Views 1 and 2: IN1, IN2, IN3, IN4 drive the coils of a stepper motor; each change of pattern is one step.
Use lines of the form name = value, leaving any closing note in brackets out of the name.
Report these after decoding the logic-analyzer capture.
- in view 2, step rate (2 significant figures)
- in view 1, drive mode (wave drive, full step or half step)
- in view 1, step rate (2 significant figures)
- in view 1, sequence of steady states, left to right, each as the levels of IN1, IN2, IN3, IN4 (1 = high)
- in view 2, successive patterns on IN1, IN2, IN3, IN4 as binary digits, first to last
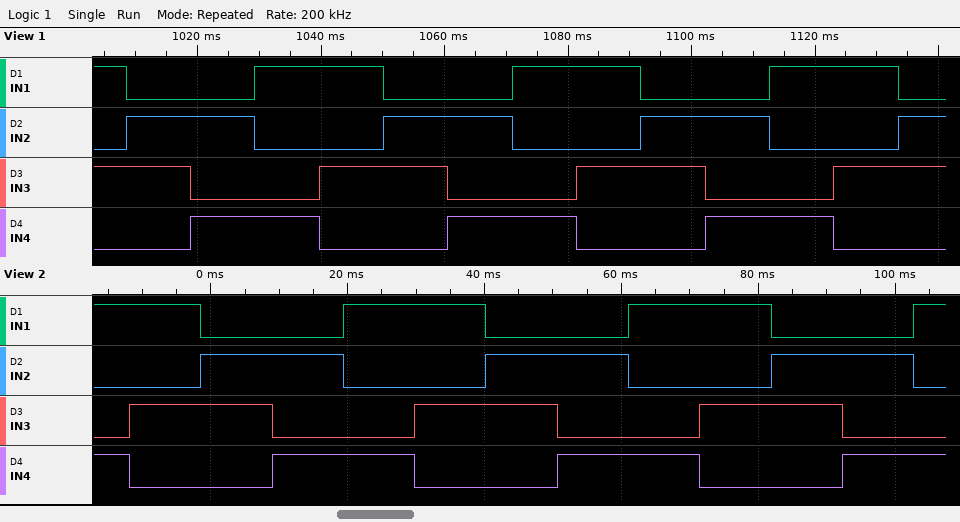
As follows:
in view 2, step rate = 96 steps/s
in view 1, drive mode = full step
in view 1, step rate = 96 steps/s
in view 1, sequence of steady states, left to right, each as the levels of IN1, IN2, IN3, IN4 = 1010 0110 0101 1001 1010 0110 0101 1001 1010 0110 0101 1001 1010 0110
in view 2, successive patterns on IN1, IN2, IN3, IN4 as binary digits, first to last = 1001 1010 0110 0101 1001 1010 0110 0101 1001 1010 0110 0101 1001
